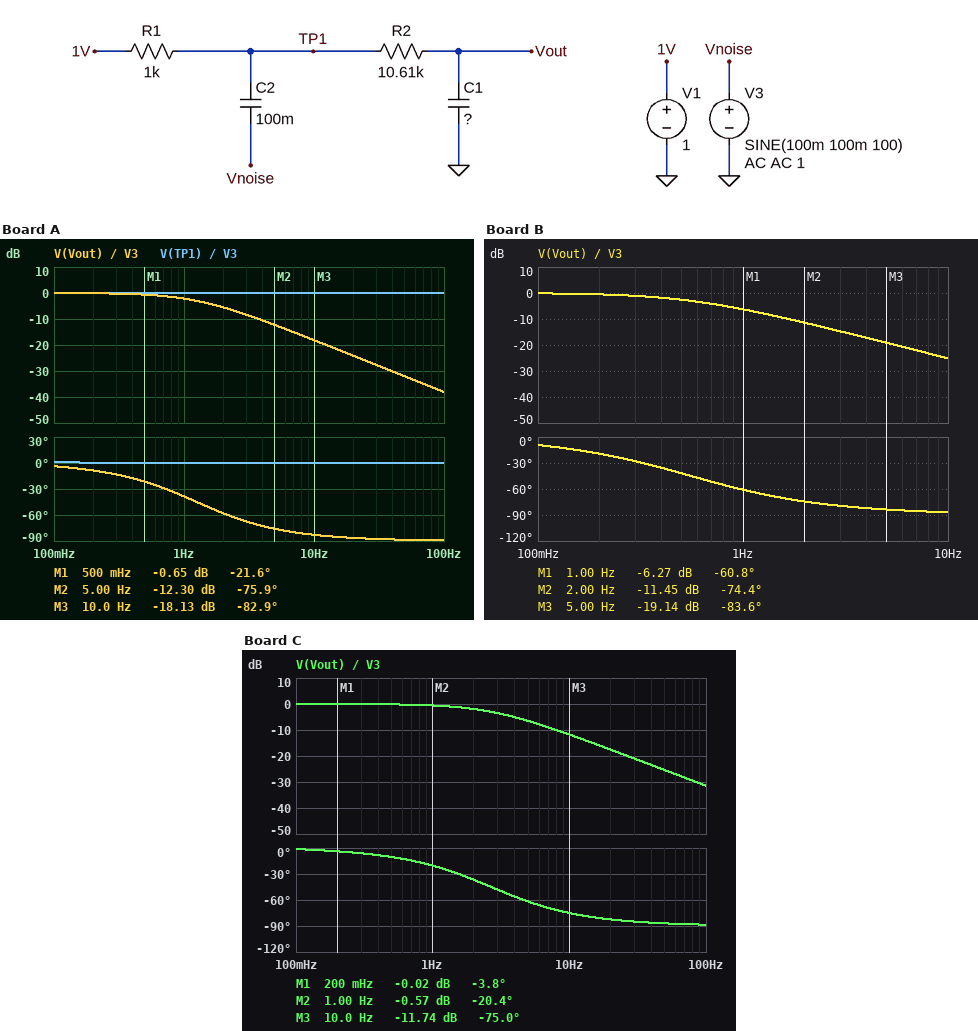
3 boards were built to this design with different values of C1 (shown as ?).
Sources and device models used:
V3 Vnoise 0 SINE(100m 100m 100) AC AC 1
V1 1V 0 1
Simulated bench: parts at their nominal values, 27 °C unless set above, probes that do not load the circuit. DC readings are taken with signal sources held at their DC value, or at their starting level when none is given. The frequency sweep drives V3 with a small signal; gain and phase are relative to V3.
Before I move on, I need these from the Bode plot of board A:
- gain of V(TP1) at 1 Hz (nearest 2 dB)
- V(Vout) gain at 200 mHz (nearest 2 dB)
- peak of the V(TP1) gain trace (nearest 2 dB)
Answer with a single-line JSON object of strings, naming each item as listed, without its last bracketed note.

{"gain of V(TP1) at 1 Hz": "0 dB", "V(Vout) gain at 200 mHz": "0 dB", "peak of the V(TP1) gain trace": "0 dB"}
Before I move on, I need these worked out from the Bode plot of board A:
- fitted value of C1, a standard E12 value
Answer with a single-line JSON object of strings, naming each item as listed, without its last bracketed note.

{"fitted value of C1, a standard E12 value": "12 µF"}
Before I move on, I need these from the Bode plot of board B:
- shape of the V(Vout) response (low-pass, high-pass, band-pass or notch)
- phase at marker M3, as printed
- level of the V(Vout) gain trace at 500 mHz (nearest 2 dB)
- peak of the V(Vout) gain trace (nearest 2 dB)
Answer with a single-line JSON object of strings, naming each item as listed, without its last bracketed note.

{"shape of the V(Vout) response": "low-pass", "phase at marker M3, as printed": "-83.6 deg", "level of the V(Vout) gain trace at 500 mHz": "-2 dB", "peak of the V(Vout) gain trace": "0 dB"}
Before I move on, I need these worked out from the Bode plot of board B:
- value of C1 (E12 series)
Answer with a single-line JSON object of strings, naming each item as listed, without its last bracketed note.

{"value of C1": "27 µF"}
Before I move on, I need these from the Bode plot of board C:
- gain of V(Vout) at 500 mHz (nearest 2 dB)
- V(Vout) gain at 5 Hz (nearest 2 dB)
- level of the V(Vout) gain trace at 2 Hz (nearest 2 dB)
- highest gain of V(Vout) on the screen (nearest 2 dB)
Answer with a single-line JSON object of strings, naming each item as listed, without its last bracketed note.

{"gain of V(Vout) at 500 mHz": "0 dB", "V(Vout) gain at 5 Hz": "-6 dB", "level of the V(Vout) gain trace at 2 Hz": "-2 dB", "highest gain of V(Vout) on the screen": "0 dB"}
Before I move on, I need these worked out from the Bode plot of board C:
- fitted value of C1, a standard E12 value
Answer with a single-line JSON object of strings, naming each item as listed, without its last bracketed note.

{"fitted value of C1, a standard E12 value": "5.6 µF"}
